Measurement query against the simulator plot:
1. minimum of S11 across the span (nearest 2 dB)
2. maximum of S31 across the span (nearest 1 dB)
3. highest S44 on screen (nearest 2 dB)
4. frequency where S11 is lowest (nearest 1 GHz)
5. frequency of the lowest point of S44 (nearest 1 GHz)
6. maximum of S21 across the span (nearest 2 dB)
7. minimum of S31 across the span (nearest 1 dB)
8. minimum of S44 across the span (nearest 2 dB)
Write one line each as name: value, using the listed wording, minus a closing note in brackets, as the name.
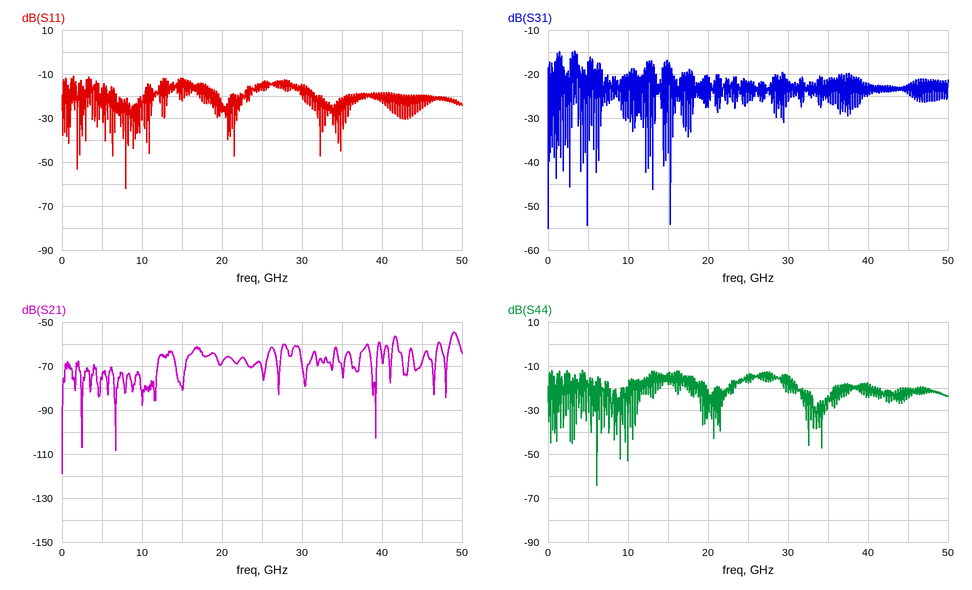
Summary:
minimum of S11 across the span: -62 dB
maximum of S31 across the span: -15 dB
highest S44 on screen: -12 dB
frequency where S11 is lowest: 8 GHz
frequency of the lowest point of S44: 6 GHz
maximum of S21 across the span: -54 dB
minimum of S31 across the span: -55 dB
minimum of S44 across the span: -64 dB
